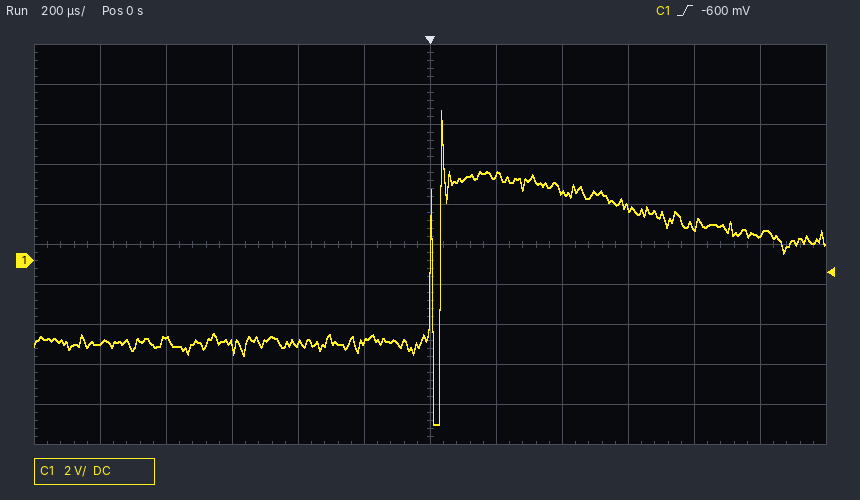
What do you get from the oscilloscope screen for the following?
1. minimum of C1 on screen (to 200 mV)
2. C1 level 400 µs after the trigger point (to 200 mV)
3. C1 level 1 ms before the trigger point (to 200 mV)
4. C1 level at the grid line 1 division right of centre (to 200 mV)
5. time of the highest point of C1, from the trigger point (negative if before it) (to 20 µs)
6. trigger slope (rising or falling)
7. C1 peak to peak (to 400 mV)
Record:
-8.2 V
3.4 V
-4.2 V
4.2 V
+40 µs
rising
15.6 V
